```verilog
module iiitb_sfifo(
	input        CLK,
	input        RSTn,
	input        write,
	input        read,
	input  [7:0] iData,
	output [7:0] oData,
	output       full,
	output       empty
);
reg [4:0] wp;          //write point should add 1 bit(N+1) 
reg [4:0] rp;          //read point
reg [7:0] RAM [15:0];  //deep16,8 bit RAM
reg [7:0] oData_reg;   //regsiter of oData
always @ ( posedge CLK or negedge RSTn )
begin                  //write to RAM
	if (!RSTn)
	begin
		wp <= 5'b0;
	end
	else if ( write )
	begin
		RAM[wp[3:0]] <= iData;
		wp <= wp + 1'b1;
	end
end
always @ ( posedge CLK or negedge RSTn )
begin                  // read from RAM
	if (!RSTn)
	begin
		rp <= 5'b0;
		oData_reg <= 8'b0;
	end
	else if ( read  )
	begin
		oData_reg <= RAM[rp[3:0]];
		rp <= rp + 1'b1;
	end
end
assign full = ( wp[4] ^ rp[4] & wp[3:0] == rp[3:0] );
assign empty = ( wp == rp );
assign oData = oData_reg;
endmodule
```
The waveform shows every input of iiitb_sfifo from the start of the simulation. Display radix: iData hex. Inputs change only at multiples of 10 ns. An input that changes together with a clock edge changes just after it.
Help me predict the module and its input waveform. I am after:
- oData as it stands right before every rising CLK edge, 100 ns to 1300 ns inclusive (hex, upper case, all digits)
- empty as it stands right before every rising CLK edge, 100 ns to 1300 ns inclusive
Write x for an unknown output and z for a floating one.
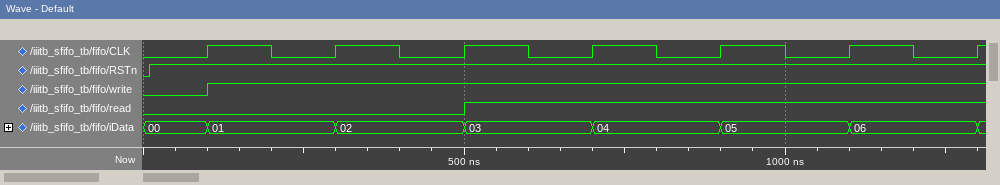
00, 00, 00, 00, 01, 02, 03
1 1 0 0 0 0 0
